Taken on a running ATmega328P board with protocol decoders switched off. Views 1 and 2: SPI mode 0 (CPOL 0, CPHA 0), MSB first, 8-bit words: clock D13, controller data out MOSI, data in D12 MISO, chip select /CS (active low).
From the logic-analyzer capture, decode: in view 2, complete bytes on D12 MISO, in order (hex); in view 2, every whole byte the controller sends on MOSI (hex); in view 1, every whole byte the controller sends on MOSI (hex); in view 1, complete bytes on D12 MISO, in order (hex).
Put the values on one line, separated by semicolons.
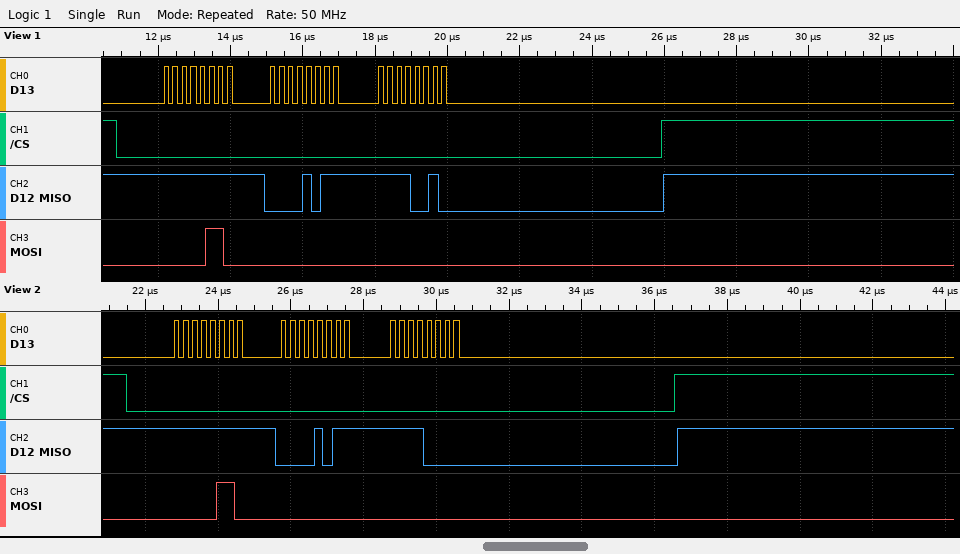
FF 0B F0; 06 00 00; 0x06 0x00 0x00; 0xFF 0x0B 0xF2
